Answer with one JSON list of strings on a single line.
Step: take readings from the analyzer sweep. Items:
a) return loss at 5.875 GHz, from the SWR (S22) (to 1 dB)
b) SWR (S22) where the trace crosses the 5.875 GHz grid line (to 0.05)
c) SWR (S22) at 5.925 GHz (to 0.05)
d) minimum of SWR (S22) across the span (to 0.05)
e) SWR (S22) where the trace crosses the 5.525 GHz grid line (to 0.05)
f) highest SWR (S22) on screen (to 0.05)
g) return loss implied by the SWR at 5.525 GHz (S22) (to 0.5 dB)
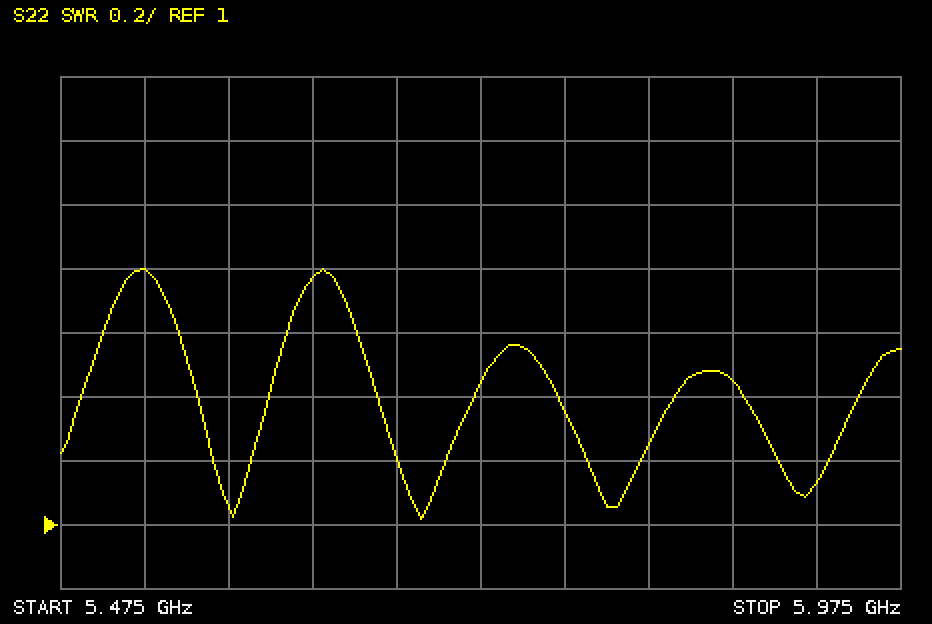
["15 dB", "1.45", "1.15", "1.00", "1.80", "1.80", "11.0 dB"]
